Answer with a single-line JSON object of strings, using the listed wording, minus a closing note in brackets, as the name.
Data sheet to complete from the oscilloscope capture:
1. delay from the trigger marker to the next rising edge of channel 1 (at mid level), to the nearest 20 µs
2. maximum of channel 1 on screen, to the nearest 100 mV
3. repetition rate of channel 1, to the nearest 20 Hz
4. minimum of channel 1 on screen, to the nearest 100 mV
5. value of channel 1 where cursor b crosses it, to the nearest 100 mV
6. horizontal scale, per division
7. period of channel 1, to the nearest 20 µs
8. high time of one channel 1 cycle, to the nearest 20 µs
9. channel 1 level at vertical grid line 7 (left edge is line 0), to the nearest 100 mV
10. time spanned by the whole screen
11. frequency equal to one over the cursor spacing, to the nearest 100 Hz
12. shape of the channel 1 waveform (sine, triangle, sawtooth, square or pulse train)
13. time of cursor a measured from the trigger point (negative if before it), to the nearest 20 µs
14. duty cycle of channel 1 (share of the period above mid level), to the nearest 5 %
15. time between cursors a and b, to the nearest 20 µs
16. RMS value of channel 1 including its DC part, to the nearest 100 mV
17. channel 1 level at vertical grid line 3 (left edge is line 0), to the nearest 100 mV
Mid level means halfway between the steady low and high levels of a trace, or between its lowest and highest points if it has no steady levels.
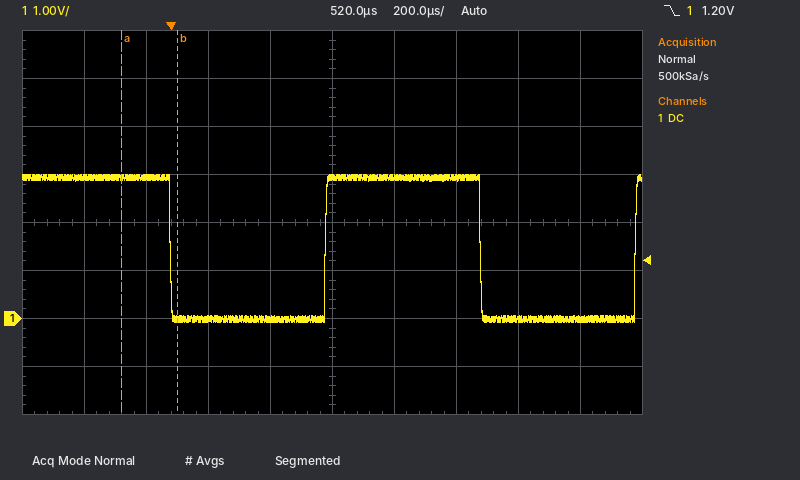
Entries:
{"delay from the trigger marker to the next rising edge of channel 1 (at mid level), to the nearest 20 µs": "500 µs", "maximum of channel 1 on screen, to the nearest 100 mV": "3.0 V", "repetition rate of channel 1, to the nearest 20 Hz": "1.00 kHz", "minimum of channel 1 on screen, to the nearest 100 mV": "-100 mV", "value of channel 1 where cursor b crosses it, to the nearest 100 mV": "0.0 V", "horizontal scale, per division": "200 µs", "period of channel 1, to the nearest 20 µs": "1.00 ms", "high time of one channel 1 cycle, to the nearest 20 µs": "500 µs", "channel 1 level at vertical grid line 7 (left edge is line 0), to the nearest 100 mV": "2.9 V", "time spanned by the whole screen": "2 ms", "frequency equal to one over the cursor spacing, to the nearest 100 Hz": "5.6 kHz", "shape of the channel 1 waveform": "square", "time of cursor a measured from the trigger point (negative if before it), to the nearest 20 µs": "-160 µs", "duty cycle of channel 1 (share of the period above mid level), to the nearest 5 %": "50 %", "time between cursors a and b, to the nearest 20 µs": "180 µs", "RMS value of channel 1 including its DC part, to the nearest 100 mV": "2.1 V", "channel 1 level at vertical grid line 3 (left edge is line 0), to the nearest 100 mV": "0.0 V"}
